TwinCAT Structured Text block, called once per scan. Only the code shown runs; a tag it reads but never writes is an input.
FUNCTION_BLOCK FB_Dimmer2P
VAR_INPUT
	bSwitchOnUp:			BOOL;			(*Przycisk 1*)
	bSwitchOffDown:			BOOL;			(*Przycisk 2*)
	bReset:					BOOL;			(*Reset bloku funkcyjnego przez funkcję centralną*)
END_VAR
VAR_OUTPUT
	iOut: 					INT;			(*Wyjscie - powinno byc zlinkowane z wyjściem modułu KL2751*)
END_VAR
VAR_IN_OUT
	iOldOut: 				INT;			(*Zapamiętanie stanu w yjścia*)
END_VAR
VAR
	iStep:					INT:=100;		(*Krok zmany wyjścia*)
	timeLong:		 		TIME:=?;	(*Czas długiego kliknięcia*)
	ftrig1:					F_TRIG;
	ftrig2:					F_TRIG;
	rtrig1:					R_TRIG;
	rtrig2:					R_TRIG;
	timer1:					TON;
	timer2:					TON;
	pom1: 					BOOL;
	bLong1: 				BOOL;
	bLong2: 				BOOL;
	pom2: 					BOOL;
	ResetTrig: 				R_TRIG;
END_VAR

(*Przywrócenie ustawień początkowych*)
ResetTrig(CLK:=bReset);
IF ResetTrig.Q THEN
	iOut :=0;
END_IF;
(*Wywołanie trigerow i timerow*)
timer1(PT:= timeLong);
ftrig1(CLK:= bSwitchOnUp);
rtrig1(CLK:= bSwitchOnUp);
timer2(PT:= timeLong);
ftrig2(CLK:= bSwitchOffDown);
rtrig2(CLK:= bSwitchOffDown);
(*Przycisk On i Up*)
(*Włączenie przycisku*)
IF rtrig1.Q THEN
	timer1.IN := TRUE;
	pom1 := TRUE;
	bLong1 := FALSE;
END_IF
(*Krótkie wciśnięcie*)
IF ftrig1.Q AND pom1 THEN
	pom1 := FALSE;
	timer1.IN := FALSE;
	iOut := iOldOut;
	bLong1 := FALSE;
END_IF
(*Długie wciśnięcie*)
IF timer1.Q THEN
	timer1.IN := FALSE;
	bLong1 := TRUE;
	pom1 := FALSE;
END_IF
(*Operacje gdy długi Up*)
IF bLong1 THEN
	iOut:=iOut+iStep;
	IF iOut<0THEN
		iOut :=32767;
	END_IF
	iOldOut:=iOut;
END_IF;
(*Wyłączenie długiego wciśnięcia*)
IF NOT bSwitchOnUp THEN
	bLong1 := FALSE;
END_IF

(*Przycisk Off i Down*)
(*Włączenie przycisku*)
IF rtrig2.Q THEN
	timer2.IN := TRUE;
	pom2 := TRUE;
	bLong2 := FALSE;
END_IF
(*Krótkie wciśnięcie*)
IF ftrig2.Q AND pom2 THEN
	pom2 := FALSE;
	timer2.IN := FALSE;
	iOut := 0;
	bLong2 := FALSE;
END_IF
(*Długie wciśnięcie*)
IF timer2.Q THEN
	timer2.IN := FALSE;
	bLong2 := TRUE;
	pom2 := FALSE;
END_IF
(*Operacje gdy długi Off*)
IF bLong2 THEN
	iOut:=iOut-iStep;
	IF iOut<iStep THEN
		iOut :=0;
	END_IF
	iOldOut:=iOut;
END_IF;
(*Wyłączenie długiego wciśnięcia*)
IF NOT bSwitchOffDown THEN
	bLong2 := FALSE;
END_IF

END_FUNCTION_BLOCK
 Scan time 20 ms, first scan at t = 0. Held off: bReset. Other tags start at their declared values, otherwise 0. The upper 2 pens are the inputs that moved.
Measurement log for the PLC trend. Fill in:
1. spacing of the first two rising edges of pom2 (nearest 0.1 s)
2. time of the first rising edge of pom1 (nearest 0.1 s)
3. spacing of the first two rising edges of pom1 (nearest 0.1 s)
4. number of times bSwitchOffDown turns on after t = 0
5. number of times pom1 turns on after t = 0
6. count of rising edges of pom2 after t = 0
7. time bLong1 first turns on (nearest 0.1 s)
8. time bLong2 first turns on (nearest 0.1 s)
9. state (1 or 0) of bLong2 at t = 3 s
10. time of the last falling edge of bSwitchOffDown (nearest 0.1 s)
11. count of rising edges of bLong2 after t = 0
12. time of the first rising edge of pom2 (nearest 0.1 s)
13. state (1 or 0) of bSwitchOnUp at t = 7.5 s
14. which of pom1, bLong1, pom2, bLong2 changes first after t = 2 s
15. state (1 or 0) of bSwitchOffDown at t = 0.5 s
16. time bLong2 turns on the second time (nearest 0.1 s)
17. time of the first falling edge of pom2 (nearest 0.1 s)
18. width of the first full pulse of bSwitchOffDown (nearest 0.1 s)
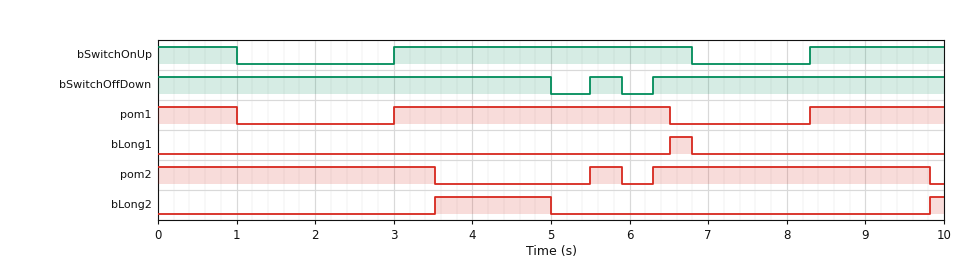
0.8 s
3.0 s
5.3 s
2
2
2
6.5 s
3.5 s
0
5.9 s
2
5.5 s
0
pom1
1
9.8 s
3.5 s
0.4 s
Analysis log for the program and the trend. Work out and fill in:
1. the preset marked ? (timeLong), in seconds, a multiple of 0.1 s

3.5 s
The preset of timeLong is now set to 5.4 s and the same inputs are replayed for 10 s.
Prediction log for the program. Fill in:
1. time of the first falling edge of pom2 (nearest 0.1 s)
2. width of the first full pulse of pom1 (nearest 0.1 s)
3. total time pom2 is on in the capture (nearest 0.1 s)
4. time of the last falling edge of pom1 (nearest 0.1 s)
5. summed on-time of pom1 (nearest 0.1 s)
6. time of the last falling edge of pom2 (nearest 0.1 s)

5.0 s
3.8 s
9.1 s
6.8 s
6.5 s
5.9 s
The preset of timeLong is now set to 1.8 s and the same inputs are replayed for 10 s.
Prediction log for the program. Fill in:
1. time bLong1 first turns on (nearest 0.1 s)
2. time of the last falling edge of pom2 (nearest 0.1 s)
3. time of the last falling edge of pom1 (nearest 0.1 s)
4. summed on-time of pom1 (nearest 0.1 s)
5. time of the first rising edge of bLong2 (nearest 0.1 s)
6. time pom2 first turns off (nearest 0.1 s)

4.8 s
8.1 s
4.8 s
4.5 s
1.8 s
1.8 s
